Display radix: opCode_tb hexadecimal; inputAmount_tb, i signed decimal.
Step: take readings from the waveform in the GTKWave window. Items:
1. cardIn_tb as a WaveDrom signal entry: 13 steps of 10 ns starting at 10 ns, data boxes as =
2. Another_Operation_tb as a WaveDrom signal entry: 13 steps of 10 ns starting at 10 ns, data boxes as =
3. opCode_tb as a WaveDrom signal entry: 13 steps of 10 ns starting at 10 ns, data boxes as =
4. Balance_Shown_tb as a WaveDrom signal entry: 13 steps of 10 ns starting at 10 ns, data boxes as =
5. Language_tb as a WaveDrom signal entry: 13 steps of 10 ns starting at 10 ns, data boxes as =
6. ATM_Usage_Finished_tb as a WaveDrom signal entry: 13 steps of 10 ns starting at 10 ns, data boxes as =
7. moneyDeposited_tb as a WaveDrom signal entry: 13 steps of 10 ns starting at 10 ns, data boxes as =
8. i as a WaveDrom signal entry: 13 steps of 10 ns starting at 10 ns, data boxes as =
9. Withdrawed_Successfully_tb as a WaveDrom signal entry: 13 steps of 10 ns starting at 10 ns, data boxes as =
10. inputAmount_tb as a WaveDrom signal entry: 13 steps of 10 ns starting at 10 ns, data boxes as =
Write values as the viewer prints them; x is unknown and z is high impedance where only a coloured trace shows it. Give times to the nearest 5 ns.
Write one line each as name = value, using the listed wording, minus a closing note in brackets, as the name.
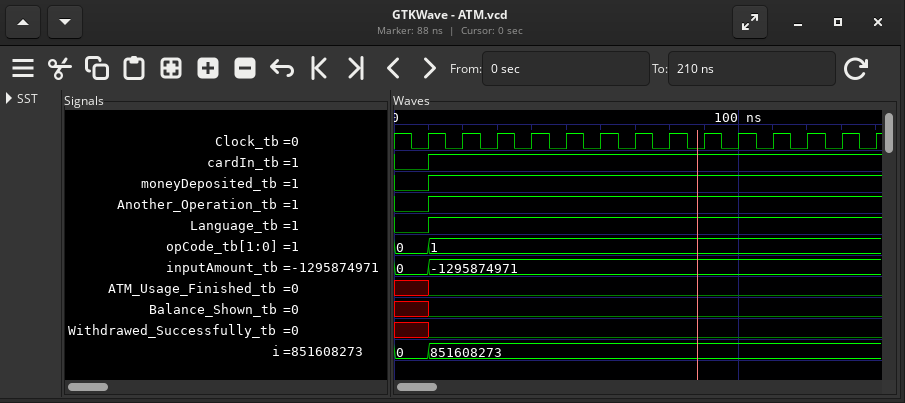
cardIn_tb as a WaveDrom signal entry: 13 steps of 10 ns starting at 10 ns, data boxes as = = {name: 'cardIn_tb', wave: '1............'}
Another_Operation_tb as a WaveDrom signal entry: 13 steps of 10 ns starting at 10 ns, data boxes as = = {name: 'Another_Operation_tb', wave: '1............'}
opCode_tb as a WaveDrom signal entry: 13 steps of 10 ns starting at 10 ns, data boxes as = = {name: 'opCode_tb', wave: '=............', data: '1'}
Balance_Shown_tb as a WaveDrom signal entry: 13 steps of 10 ns starting at 10 ns, data boxes as = = {name: 'Balance_Shown_tb', wave: '0............'}
Language_tb as a WaveDrom signal entry: 13 steps of 10 ns starting at 10 ns, data boxes as = = {name: 'Language_tb', wave: '1............'}
ATM_Usage_Finished_tb as a WaveDrom signal entry: 13 steps of 10 ns starting at 10 ns, data boxes as = = {name: 'ATM_Usage_Finished_tb', wave: '0............'}
moneyDeposited_tb as a WaveDrom signal entry: 13 steps of 10 ns starting at 10 ns, data boxes as = = {name: 'moneyDeposited_tb', wave: '1............'}
i as a WaveDrom signal entry: 13 steps of 10 ns starting at 10 ns, data boxes as = = {name: 'i', wave: '=............', data: '851608273'}
Withdrawed_Successfully_tb as a WaveDrom signal entry: 13 steps of 10 ns starting at 10 ns, data boxes as = = {name: 'Withdrawed_Successfully_tb', wave: '0............'}
inputAmount_tb as a WaveDrom signal entry: 13 steps of 10 ns starting at 10 ns, data boxes as = = {name: 'inputAmount_tb', wave: '=............', data: '-1295874971'}
